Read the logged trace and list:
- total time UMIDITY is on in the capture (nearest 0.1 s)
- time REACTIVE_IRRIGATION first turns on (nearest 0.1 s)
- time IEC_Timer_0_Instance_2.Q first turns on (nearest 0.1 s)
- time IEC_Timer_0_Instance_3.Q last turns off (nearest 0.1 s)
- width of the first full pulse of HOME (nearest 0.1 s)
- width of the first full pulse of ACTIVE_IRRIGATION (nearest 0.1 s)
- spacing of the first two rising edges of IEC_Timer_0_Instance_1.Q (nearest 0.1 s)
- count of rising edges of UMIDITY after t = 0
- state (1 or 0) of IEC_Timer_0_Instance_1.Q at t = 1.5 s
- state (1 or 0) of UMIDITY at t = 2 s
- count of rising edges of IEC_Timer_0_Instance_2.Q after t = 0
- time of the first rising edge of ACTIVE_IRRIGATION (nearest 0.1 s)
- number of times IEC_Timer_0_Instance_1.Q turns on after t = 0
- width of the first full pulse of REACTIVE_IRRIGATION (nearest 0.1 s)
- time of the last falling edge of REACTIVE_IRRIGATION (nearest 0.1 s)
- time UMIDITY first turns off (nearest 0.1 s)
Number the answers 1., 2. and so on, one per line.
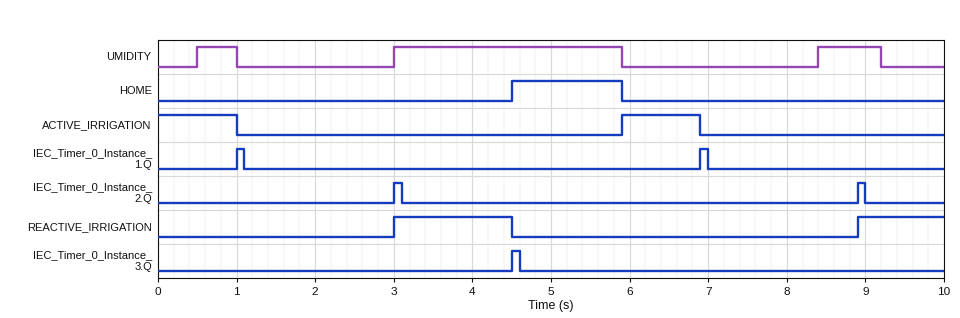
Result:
1. 4.2 s
2. 3.0 s
3. 3.0 s
4. 4.6 s
5. 1.4 s
6. 1.0 s
7. 5.9 s
8. 3
9. 0
10. 0
11. 2
12. 5.9 s
13. 2
14. 1.5 s
15. 4.5 s
16. 1.0 s
